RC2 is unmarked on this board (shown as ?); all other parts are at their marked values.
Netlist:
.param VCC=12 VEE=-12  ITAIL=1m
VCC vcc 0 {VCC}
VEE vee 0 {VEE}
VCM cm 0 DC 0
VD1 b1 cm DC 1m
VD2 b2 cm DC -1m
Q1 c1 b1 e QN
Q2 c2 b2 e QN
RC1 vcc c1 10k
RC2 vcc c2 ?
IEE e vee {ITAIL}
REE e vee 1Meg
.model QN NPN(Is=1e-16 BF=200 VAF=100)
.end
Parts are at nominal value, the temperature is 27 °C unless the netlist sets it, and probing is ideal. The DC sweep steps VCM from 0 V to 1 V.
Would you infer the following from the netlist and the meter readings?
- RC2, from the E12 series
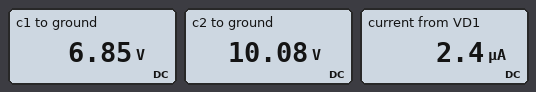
3.9 kΩ
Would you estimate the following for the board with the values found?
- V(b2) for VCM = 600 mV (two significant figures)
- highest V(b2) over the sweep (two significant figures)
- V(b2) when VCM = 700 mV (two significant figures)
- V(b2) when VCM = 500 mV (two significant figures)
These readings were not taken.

600 mV
1.0 V
700 mV
500 mV
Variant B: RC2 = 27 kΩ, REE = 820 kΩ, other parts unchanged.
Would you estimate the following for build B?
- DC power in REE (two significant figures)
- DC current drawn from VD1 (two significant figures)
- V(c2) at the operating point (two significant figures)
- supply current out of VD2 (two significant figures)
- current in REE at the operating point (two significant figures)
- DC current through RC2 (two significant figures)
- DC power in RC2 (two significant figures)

150 µW
2.5 µA
-590 mV
3.1 µA
14 µA
470 µA
5.9 mW
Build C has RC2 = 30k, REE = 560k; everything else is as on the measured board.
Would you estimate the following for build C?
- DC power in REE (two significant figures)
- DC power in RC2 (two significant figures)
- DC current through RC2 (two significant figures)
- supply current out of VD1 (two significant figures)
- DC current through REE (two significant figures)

230 µW
5.4 mW
420 µA
2.6 µA
20 µA
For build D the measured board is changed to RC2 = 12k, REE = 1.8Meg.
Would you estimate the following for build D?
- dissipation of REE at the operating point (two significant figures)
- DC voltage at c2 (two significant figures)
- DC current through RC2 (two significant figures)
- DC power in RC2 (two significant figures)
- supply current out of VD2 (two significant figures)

70 µW
6.2 V
480 µA
2.8 mW
2.3 µA
